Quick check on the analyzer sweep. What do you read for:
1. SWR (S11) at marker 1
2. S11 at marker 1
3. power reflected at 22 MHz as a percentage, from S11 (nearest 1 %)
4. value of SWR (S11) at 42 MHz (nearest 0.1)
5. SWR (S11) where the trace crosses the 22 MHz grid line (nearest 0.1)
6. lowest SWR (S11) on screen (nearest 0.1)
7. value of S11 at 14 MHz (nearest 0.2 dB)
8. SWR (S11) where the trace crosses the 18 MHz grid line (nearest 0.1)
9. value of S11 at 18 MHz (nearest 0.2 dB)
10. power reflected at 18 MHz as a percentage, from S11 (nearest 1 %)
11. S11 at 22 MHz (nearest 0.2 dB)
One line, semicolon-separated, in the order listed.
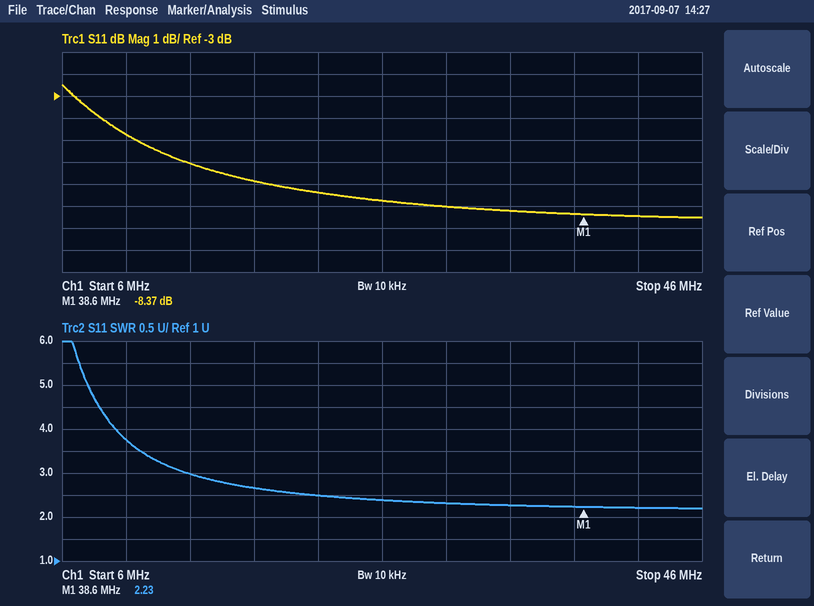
2.23; -8.37 dB; 18 %; 2.2; 2.5; 2.2; -6.0 dB; 2.7; -6.8 dB; 21 %; -7.4 dB
